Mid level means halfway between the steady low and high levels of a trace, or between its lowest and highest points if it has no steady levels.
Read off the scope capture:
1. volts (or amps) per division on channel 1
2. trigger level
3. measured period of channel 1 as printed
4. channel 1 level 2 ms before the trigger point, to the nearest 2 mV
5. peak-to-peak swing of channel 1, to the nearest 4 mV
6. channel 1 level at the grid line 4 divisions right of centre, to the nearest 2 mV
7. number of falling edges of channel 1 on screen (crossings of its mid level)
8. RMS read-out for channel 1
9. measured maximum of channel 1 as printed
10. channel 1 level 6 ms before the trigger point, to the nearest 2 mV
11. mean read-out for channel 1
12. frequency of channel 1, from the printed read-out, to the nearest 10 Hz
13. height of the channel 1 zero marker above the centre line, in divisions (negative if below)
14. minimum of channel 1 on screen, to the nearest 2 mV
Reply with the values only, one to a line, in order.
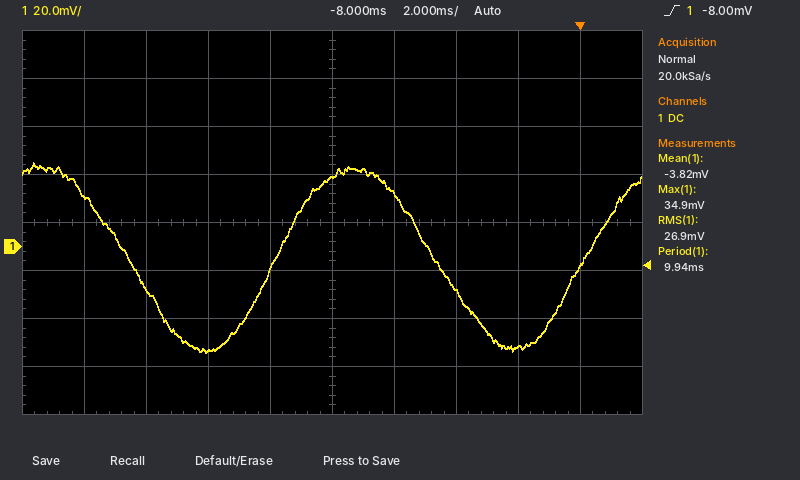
20 mV
-8.00 mV
9.94 ms
-42 mV
80 mV
-8 mV
2
26.9 mV
34.9 mV
22 mV
-3.82 mV
100 Hz
-0.5 div
-44 mV
